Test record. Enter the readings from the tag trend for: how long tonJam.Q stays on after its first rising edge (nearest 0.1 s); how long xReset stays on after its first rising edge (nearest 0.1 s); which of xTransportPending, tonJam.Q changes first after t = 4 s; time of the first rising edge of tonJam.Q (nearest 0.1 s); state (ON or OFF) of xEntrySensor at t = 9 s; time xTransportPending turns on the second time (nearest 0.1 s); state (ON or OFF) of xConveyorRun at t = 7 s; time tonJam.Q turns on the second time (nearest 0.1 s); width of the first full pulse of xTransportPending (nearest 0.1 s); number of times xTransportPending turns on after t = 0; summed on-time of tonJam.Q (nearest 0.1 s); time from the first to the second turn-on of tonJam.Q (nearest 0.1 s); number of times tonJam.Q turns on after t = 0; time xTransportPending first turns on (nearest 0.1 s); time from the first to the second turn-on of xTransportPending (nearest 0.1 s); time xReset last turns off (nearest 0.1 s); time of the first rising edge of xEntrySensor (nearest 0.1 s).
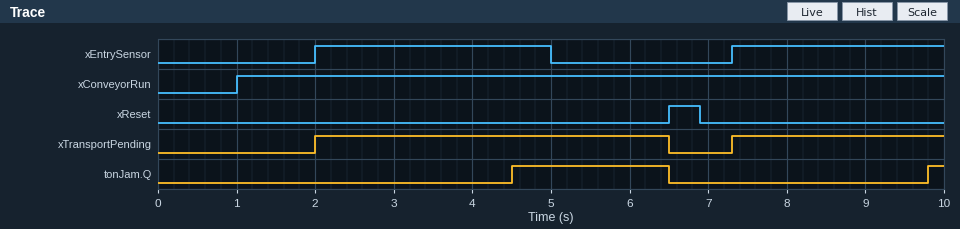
2.0 s
0.4 s
tonJam.Q
4.5 s
ON
7.3 s
ON
9.8 s
4.5 s
2
2.2 s
5.3 s
2
2.0 s
5.3 s
6.9 s
2.0 s
